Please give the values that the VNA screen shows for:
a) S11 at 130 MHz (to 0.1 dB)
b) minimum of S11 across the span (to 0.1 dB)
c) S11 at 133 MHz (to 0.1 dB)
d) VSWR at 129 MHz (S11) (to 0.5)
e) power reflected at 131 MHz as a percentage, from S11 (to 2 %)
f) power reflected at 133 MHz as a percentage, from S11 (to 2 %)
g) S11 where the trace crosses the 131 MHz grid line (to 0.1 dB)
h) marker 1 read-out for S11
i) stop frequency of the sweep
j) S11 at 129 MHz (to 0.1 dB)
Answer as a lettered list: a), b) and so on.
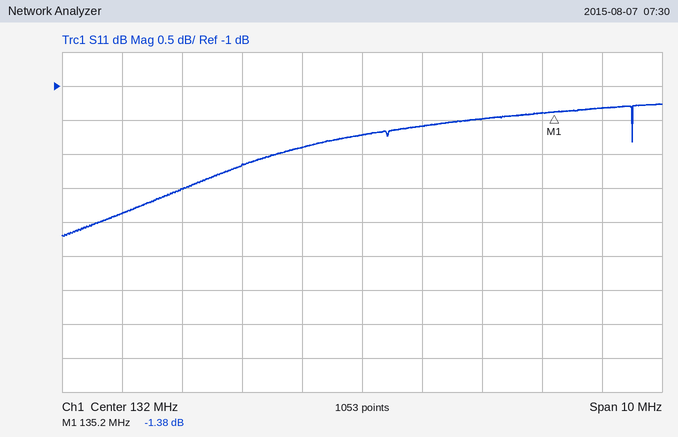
a) -2.2 dB
b) -3.2 dB
c) -1.6 dB
d) 7.0
e) 64 %
f) 70 %
g) -1.9 dB
h) -1.38 dB
i) 137 MHz
j) -2.5 dB
